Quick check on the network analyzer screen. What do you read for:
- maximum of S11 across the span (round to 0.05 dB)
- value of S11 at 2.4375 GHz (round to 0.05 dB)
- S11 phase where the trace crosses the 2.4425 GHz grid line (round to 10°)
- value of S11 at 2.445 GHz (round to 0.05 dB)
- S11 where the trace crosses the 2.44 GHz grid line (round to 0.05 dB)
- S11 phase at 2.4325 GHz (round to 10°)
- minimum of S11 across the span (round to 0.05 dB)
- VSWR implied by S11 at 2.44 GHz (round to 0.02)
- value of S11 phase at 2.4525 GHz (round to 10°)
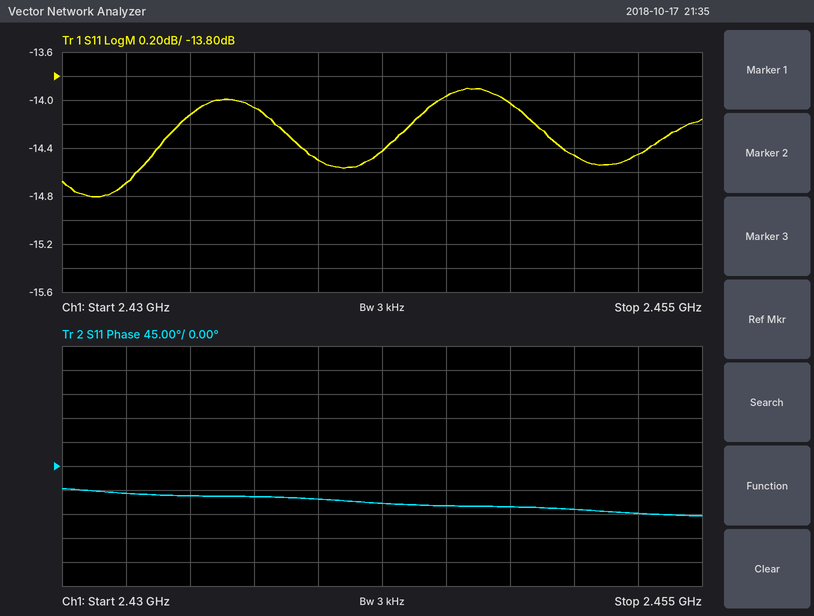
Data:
-13.90 dB
-14.05 dB
-70°
-13.95 dB
-14.50 dB
-50°
-14.80 dB
1.46
-90°
